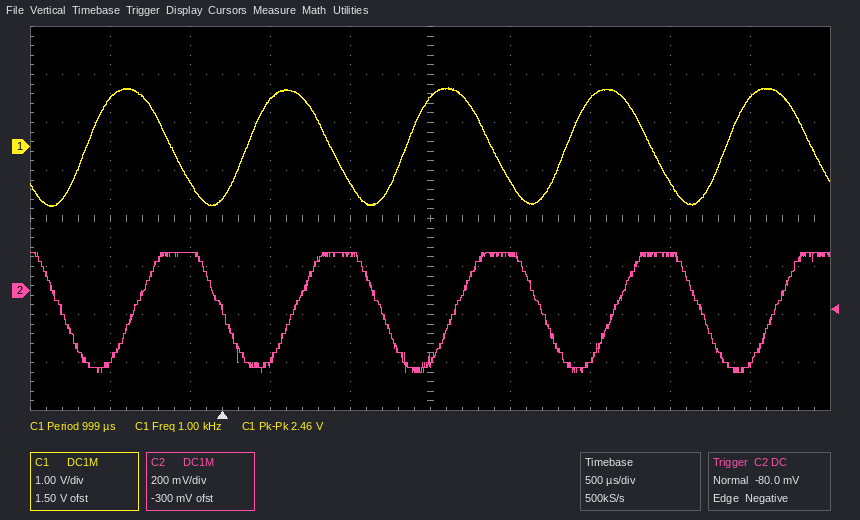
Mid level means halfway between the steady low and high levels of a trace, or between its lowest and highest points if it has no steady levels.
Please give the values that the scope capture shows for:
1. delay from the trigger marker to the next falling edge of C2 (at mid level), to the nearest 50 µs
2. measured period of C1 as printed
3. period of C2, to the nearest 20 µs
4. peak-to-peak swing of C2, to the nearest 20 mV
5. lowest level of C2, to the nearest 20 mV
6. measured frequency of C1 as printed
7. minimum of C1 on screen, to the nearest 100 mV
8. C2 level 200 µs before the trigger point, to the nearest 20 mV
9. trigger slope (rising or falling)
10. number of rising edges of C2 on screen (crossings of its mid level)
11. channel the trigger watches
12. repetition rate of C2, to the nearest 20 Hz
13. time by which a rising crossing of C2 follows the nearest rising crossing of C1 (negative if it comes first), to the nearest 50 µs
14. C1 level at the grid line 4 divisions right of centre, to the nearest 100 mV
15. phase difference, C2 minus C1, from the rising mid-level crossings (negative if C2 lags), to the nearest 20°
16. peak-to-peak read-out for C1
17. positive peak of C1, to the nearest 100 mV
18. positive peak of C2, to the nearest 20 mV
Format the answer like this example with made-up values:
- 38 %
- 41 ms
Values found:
- 1.00 ms
- 999 µs
- 1.00 ms
- 500 mV
- -340 mV
- 1.00 kHz
- -1.2 V
- 160 mV
- falling
- 5
- C2
- 1.00 kHz
- +300 µs
- 1.0 V
- -100°
- 2.46 V
- 1.2 V
- 160 mV
